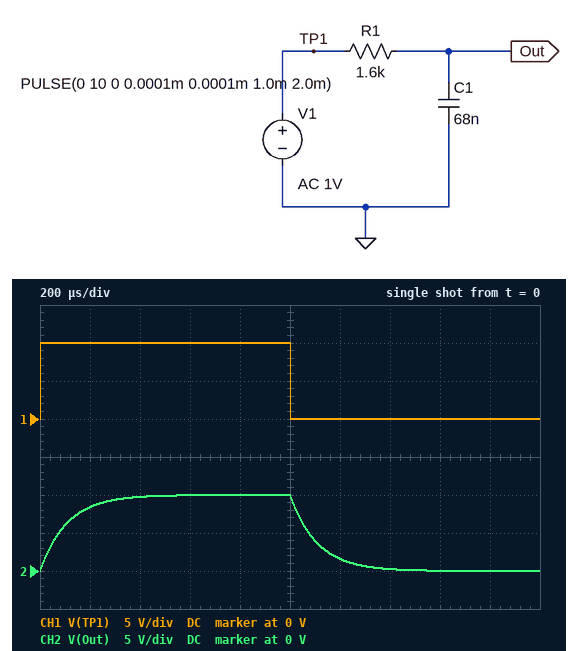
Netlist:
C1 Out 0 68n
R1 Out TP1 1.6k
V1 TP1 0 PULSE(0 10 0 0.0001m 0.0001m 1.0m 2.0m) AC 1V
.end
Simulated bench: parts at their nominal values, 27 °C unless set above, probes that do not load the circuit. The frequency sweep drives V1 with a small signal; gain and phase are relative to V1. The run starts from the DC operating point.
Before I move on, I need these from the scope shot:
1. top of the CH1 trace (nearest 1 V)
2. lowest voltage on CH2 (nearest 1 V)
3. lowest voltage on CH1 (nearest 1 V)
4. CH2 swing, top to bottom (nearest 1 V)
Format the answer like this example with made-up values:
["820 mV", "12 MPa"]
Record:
["10 V", "0 V", "0 V", "10 V"]
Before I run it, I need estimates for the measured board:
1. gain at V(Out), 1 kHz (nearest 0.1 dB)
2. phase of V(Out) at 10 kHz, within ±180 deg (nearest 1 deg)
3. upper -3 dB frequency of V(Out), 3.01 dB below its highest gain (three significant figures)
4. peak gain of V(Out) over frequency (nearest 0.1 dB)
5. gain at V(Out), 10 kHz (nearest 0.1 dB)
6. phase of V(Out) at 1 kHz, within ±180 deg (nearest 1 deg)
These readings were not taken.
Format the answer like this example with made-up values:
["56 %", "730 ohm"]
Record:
["-1.7 dB", "-82 deg", "1.46 kHz", "0 dB", "-16.8 dB", "-34 deg"]
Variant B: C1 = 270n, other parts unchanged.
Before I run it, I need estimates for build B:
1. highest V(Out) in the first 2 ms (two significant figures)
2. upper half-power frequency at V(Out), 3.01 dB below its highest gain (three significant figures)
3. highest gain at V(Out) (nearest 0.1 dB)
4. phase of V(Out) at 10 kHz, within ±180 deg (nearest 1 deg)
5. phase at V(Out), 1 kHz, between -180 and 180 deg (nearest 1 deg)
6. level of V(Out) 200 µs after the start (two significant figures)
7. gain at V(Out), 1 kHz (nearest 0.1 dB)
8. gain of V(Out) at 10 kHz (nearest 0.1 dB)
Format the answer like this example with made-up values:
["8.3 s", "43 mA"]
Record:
["9.0 V", "368 Hz", "0 dB", "-88 deg", "-70 deg", "3.7 V", "-9.2 dB", "-28.7 dB"]
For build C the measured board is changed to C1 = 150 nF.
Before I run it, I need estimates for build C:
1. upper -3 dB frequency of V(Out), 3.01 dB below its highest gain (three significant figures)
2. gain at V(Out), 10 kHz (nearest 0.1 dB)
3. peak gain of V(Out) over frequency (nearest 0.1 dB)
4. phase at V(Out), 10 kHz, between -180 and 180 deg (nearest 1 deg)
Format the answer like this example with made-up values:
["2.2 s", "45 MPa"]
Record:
["663 Hz", "-23.6 dB", "0 dB", "-86 deg"]
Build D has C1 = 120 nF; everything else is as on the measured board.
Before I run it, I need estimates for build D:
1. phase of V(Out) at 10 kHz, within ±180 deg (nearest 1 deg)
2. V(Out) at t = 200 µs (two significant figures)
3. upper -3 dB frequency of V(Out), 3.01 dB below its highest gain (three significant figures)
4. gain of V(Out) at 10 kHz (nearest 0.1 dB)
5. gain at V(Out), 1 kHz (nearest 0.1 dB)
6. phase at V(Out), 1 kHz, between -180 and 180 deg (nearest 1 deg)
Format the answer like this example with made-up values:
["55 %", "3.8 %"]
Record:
["-85 deg", "6.5 V", "829 Hz", "-21.7 dB", "-3.9 dB", "-50 deg"]
